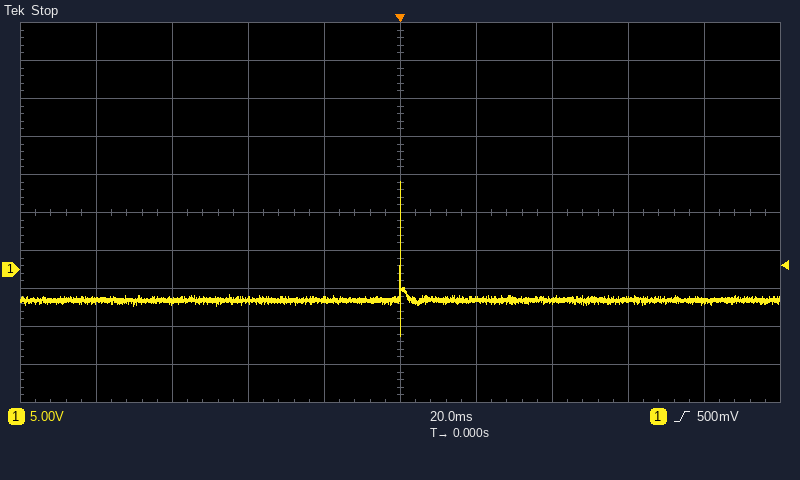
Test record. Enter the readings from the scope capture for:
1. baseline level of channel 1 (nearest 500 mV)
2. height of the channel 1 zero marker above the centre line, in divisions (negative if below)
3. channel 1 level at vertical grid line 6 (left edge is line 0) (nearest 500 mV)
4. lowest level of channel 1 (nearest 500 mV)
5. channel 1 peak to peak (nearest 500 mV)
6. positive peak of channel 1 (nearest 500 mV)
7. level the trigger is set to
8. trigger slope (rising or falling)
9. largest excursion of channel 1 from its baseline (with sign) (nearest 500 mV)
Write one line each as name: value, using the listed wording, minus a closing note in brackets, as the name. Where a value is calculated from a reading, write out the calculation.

baseline level of channel 1: -4.0 V
height of the channel 1 zero marker above the centre line, in divisions: -1.5 div
channel 1 level at vertical grid line 6 (left edge is line 0): -4.0 V
lowest level of channel 1: -9.0 V
channel 1 peak to peak: 11.5 V − (-9.0 V) = 20.5 V
positive peak of channel 1: 11.5 V
level the trigger is set to: 500 mV
trigger slope: rising
largest excursion of channel 1 from its baseline (with sign): 11.5 V − (-4.0 V) = +15.5 V
